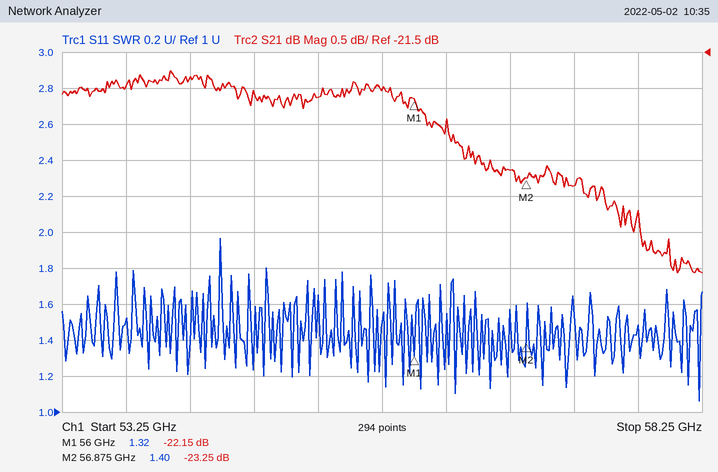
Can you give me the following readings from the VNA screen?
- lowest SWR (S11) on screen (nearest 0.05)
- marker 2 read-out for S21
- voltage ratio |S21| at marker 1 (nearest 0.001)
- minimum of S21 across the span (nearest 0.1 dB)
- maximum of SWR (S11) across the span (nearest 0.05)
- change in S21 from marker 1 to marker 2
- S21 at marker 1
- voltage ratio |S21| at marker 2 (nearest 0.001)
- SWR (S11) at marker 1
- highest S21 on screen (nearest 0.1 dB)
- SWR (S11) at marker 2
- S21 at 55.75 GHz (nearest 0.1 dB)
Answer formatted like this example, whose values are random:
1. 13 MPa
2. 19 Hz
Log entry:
1. 1.05
2. -23.25 dB
3. 0.078
4. -24.6 dB
5. 1.95
6. -1.10 dB
7. -22.15 dB
8. 0.069
9. 1.32
10. -21.8 dB
11. 1.40
12. -22.0 dB
